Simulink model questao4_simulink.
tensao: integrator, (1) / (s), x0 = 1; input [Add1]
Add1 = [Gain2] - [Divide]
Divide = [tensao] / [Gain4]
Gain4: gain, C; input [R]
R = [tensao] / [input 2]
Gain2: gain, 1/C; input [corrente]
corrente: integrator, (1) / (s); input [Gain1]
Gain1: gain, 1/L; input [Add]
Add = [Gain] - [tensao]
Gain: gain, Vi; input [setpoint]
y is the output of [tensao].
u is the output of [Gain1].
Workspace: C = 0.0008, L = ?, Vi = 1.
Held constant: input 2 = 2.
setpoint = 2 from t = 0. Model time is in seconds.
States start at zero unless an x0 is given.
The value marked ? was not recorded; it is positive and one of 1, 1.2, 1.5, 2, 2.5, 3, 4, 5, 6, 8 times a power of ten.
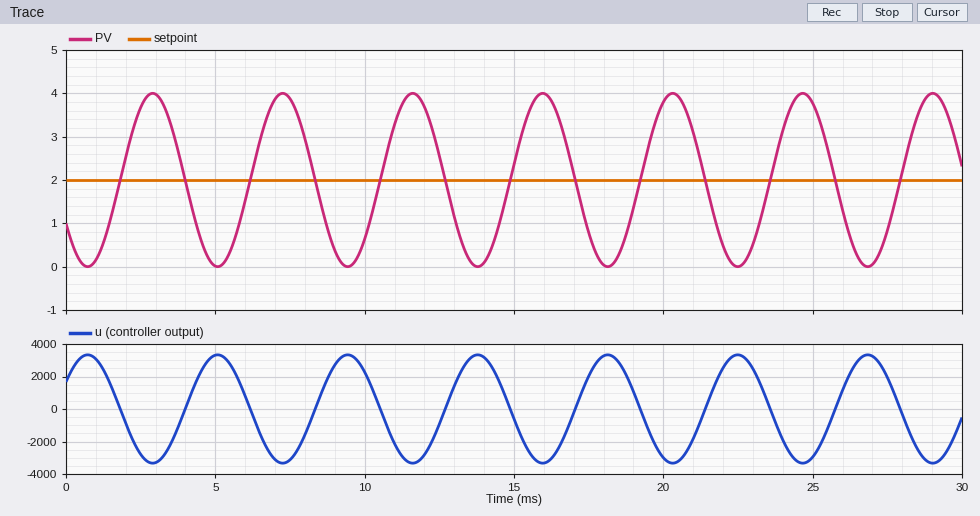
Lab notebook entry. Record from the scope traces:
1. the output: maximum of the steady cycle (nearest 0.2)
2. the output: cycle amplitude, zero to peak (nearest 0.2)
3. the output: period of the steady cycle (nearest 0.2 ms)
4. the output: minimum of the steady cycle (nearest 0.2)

4.0
2.0
4.4 ms
0.0
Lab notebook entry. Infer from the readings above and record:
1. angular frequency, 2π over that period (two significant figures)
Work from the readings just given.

1.4 rad/ms
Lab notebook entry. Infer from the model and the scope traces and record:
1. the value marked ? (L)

0.0006
